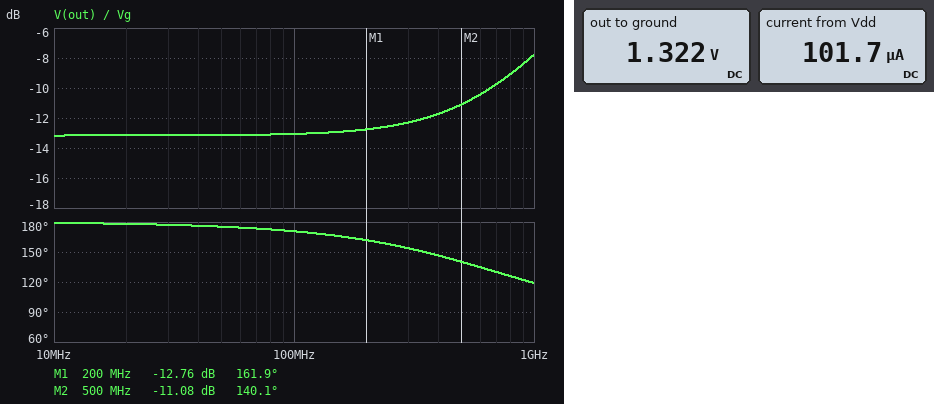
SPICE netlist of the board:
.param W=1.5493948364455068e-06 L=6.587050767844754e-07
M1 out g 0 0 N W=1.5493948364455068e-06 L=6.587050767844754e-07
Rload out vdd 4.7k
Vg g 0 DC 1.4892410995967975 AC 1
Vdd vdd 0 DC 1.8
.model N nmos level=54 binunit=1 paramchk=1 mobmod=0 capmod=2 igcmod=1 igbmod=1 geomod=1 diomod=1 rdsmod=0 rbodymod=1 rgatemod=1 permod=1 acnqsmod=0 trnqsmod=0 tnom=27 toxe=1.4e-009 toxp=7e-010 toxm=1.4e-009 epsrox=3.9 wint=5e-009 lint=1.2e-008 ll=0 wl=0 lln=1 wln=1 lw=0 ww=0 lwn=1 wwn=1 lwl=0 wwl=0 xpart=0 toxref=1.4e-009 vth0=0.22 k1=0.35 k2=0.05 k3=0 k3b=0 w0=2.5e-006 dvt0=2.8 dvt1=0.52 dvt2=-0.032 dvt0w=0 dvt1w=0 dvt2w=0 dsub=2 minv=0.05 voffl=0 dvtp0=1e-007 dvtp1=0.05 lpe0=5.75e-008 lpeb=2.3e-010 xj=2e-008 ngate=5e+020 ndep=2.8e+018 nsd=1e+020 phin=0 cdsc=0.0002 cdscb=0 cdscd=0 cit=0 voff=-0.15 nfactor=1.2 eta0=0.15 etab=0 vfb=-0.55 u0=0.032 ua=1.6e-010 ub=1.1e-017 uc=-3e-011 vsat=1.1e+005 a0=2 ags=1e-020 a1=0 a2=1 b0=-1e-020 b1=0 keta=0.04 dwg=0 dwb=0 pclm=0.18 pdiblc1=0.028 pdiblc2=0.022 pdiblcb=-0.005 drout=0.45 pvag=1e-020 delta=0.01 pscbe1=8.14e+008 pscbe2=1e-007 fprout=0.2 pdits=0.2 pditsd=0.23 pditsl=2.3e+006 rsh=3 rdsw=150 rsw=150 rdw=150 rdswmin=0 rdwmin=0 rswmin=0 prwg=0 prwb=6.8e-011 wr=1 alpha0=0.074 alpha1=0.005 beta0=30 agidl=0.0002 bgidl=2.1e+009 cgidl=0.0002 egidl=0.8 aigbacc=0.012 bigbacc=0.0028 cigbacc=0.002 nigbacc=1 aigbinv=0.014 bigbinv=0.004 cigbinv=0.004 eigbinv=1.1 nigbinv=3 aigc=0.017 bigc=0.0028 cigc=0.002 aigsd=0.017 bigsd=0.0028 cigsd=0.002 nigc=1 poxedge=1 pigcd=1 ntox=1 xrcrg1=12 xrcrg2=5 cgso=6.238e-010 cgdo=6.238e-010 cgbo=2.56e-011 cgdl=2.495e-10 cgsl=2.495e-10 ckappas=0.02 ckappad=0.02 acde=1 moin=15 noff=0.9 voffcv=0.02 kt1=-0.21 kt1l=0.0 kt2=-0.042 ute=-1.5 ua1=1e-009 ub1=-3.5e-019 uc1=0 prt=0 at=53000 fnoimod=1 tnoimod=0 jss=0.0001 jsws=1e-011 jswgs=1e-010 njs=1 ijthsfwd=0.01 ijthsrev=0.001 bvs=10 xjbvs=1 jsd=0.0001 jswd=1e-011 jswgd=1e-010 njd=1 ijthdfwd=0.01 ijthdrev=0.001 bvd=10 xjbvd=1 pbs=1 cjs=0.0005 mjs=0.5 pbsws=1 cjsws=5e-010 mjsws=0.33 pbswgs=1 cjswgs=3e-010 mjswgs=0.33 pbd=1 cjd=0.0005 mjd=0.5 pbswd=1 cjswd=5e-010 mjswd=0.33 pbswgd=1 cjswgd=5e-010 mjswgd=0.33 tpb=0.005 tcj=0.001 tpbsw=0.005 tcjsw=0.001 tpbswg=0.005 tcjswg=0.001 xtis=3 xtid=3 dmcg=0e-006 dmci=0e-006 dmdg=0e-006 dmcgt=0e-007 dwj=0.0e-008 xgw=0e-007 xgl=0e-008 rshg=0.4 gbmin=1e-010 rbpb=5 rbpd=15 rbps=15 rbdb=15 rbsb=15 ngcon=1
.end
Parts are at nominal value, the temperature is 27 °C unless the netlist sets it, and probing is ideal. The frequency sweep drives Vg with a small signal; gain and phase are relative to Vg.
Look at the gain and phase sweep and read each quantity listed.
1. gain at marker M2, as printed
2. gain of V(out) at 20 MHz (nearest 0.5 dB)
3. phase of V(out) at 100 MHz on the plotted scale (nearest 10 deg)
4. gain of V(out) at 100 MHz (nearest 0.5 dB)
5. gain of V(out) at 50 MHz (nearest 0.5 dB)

-11.08 dB
-13.0 dB
170 deg
-13.0 dB
-13.0 dB
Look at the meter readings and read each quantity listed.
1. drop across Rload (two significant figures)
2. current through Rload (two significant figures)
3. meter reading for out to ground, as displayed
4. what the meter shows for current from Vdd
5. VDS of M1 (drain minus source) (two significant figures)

480 mV
100 µA
1.322 V
101.7 µA
1.3 V
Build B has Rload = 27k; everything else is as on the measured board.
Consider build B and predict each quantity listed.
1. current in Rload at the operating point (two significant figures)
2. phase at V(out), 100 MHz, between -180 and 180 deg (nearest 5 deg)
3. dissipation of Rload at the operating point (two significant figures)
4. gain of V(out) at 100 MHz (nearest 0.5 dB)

55 µA
75 deg
83 µW
-23.0 dB
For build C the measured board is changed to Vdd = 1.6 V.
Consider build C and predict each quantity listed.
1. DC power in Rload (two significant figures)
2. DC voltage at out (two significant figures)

47 µW
1.1 V
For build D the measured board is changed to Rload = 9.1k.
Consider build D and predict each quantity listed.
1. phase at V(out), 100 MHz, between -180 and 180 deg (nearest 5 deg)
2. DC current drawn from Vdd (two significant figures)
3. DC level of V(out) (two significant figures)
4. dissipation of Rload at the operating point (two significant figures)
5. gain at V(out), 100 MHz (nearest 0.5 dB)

170 deg
98 µA
910 mV
87 µW
-8.5 dB
